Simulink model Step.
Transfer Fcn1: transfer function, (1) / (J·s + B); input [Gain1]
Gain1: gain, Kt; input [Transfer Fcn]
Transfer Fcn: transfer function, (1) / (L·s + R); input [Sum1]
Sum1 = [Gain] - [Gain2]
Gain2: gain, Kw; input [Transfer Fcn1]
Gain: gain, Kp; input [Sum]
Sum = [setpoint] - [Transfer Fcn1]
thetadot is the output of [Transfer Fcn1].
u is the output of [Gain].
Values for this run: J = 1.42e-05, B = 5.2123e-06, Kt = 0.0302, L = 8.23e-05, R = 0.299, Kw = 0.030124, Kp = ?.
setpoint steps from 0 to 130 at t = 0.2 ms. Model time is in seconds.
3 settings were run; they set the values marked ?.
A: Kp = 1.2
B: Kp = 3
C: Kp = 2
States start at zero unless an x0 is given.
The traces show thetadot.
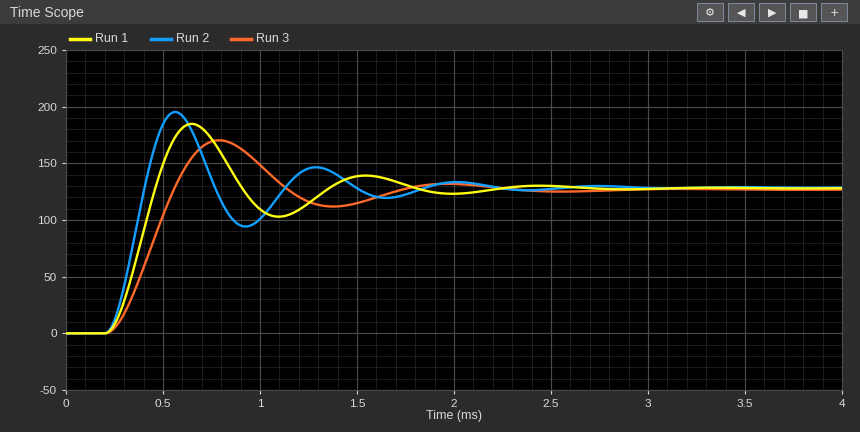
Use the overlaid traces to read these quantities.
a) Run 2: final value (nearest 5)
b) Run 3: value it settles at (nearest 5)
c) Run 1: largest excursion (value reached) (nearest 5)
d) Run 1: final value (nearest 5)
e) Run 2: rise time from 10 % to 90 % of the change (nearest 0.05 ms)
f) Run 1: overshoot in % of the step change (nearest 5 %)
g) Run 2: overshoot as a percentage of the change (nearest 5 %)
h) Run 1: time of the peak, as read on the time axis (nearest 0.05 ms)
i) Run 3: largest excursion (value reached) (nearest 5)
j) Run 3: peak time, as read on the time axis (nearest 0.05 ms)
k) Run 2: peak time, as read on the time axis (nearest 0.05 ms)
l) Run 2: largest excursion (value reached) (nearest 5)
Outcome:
130
125
185
130
0.15 ms
45 %
50 %
0.65 ms
170
0.80 ms
0.55 ms
195
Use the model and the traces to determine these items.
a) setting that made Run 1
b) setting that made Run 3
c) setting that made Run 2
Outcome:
C
A
B
